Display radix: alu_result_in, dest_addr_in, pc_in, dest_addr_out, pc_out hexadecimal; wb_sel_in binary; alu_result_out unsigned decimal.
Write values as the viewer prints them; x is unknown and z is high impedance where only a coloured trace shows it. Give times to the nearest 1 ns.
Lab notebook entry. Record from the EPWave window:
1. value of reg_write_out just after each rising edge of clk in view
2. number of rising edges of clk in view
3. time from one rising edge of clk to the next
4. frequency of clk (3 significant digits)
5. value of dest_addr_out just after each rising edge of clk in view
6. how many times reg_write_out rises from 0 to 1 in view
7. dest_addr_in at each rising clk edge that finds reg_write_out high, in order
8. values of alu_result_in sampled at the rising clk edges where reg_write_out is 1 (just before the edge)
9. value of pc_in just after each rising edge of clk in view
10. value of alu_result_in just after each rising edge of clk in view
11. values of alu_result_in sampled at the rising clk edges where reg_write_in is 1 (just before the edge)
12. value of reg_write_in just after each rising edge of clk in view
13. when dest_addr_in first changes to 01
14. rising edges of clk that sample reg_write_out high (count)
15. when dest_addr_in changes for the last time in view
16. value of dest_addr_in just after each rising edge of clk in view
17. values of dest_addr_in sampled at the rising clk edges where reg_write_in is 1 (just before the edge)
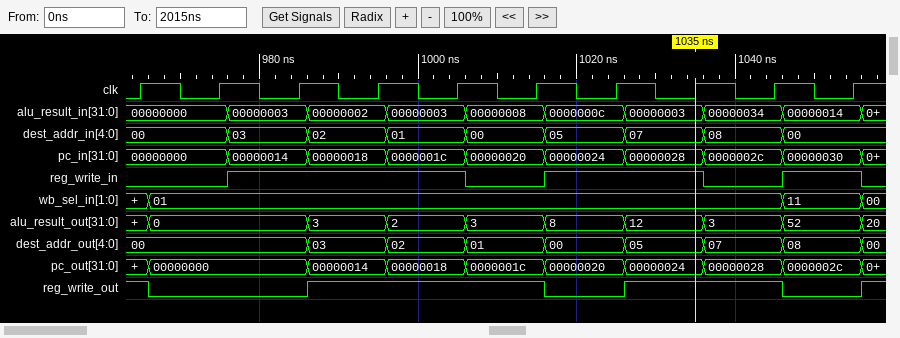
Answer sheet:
1 0 0 1 1 1 0 1 1 0
10
10 ns
100 MHz
00, 00, 00, 03, 02, 01, 00, 05, 07, 08
3
00, 02, 01, 00, 07, 08
00000000, 00000002, 00000003, 00000008, 00000003, 00000034
00000000, 00000000, 00000014, 00000018, 0000001c, 00000020, 00000024, 00000028, 0000002c, 00000030
00000000, 00000000, 00000003, 00000002, 00000003, 00000008, 0000000c, 00000003, 00000034, 00000014
00000003, 00000002, 00000003, 0000000c, 00000003, 00000014
0 0 1 1 1 0 1 1 0 1
996 ns
6
1046 ns
00, 00, 03, 02, 01, 00, 05, 07, 08, 00
03, 02, 01, 05, 07, 00
